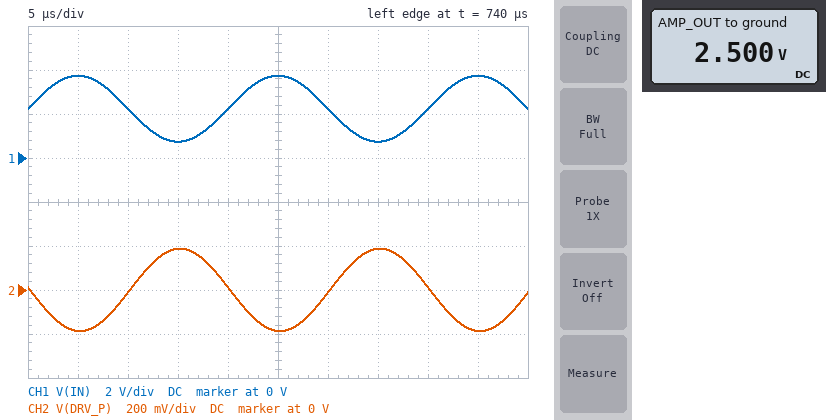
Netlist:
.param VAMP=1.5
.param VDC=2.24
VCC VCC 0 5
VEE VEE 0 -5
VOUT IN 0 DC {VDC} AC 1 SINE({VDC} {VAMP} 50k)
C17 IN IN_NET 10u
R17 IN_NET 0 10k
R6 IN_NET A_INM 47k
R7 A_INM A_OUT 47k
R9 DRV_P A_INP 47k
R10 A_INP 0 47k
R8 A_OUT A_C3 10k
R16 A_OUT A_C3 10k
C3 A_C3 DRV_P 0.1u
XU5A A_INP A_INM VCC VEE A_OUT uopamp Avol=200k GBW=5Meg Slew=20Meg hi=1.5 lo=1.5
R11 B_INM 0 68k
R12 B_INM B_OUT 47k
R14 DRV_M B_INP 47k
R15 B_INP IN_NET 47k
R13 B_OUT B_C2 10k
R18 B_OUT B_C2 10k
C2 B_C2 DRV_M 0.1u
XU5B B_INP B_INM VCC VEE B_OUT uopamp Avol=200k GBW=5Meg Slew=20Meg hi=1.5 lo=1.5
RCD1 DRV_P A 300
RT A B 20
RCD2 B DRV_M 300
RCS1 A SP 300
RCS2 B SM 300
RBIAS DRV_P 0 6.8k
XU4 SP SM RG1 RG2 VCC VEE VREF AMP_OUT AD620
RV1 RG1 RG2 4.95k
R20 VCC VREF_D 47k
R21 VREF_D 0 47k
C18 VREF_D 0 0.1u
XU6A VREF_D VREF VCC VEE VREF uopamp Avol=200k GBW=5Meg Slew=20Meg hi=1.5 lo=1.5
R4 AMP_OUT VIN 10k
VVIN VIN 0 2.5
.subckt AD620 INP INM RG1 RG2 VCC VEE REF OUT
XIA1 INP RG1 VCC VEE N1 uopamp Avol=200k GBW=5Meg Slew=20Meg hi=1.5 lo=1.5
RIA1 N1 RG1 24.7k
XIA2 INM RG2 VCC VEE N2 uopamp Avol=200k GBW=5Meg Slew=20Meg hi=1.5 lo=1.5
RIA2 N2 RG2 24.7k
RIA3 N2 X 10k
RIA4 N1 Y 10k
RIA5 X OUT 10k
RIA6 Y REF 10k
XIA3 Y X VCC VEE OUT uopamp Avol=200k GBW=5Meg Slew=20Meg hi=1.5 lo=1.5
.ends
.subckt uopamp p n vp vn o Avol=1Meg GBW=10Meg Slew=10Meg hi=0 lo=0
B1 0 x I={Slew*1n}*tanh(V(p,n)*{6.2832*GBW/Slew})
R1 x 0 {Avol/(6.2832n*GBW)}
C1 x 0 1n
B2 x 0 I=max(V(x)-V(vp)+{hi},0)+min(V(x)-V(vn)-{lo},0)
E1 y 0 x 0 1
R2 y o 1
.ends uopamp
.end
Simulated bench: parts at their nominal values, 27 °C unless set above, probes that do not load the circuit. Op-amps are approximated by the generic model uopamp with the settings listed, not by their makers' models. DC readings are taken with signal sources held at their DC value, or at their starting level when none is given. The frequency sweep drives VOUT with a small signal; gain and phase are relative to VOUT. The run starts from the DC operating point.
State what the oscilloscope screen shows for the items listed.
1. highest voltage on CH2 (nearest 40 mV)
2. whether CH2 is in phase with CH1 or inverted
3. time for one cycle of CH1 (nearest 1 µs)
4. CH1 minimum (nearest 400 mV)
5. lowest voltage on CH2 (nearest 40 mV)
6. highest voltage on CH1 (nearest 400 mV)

200 mV
inverted
20 µs
800 mV
-200 mV
3.6 V
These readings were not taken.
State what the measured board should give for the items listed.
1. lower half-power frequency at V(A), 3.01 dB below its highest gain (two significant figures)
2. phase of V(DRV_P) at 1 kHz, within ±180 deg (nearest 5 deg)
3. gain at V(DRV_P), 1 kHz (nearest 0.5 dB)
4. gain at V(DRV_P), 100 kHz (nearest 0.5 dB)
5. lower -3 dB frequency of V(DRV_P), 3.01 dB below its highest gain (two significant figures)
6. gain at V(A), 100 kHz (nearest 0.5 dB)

2.4 Hz
-155 deg
-18.5 dB
-18.0 dB
210 Hz
-23.0 dB
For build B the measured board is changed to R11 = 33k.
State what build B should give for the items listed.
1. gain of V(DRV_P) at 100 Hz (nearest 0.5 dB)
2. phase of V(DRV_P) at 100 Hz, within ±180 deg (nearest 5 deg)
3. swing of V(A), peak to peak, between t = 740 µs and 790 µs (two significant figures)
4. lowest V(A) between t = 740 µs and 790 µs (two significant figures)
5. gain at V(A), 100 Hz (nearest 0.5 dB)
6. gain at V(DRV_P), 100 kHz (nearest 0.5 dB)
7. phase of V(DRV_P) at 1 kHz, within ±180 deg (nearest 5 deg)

-19.0 dB
45 deg
1.6 V
-820 mV
-17.5 dB
-7.0 dB
20 deg
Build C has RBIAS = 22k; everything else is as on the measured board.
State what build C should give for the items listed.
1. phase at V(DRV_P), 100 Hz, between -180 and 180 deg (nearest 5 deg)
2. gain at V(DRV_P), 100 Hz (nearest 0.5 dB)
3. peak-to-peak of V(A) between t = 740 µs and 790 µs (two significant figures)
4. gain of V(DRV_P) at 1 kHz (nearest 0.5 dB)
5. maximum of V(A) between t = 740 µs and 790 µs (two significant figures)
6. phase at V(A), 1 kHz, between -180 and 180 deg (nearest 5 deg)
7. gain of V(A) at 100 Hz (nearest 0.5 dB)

-55 deg
-15.0 dB
600 mV
-12.0 dB
300 mV
-155 deg
-15.5 dB
